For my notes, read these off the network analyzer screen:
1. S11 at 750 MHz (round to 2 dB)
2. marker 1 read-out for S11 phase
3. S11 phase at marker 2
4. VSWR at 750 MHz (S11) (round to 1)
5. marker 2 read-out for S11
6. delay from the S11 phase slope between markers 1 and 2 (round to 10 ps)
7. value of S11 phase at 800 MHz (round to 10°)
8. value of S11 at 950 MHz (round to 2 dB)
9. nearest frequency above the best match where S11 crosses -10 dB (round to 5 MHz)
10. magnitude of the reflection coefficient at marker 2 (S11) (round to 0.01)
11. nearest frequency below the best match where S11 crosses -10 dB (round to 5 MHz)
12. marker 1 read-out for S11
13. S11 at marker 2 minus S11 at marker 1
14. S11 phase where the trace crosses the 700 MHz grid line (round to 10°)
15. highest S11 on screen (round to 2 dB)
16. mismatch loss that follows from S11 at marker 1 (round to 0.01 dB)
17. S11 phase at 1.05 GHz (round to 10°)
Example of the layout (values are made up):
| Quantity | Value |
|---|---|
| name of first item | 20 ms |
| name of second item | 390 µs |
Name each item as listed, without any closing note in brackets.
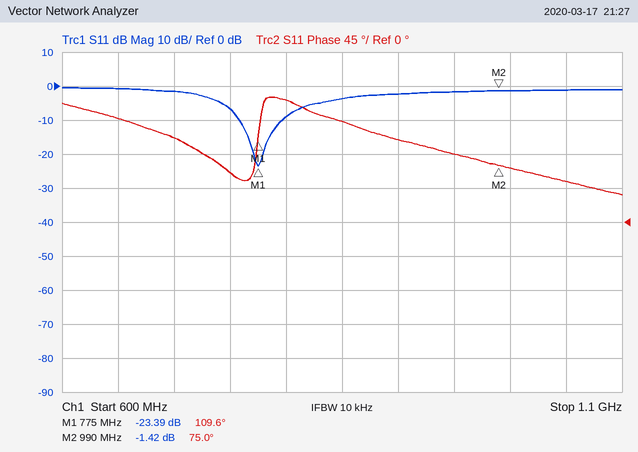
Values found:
| Quantity | Value |
|---|---|
| S11 at 750 MHz | -6 dB |
| marker 1 read-out for S11 phase | 109.6° |
| S11 phase at marker 2 | 75.0° |
| VSWR at 750 MHz (S11) | 3 |
| marker 2 read-out for S11 | -1.42 dB |
| delay from the S11 phase slope between markers 1 and 2 | 450 ps |
| value of S11 phase at 800 MHz | 160° |
| value of S11 at 950 MHz | -2 dB |
| nearest frequency above the best match where S11 crosses -10 dB | 795 MHz |
| magnitude of the reflection coefficient at marker 2 (S11) | 0.85 |
| nearest frequency below the best match where S11 crosses -10 dB | 760 MHz |
| marker 1 read-out for S11 | -23.39 dB |
| S11 at marker 2 minus S11 at marker 1 | 21.97 dB |
| S11 phase where the trace crosses the 700 MHz grid line | 110° |
| highest S11 on screen | 0 dB |
| mismatch loss that follows from S11 at marker 1 | 0.02 dB |
| S11 phase at 1.05 GHz | 50° |
